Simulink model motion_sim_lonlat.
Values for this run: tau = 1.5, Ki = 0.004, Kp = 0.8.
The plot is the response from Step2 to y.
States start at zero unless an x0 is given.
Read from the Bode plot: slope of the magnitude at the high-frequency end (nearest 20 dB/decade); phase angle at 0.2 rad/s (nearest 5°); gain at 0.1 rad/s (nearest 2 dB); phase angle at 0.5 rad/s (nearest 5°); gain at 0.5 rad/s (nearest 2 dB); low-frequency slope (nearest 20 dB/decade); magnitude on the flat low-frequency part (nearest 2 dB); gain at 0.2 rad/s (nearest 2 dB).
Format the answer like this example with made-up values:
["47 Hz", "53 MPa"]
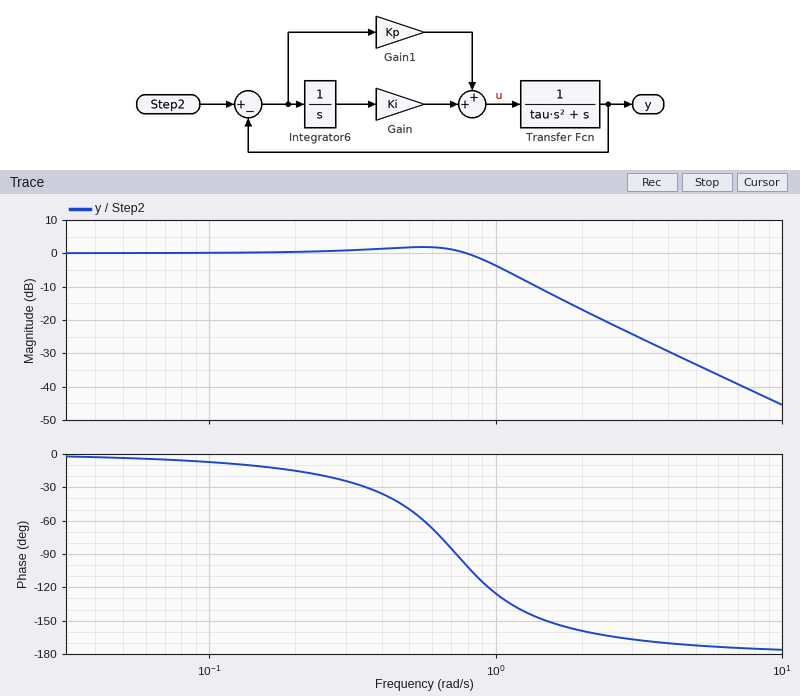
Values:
["-40 dB/decade", "-15°", "0 dB", "-50°", "2 dB", "0 dB/decade", "0 dB", "0 dB"]
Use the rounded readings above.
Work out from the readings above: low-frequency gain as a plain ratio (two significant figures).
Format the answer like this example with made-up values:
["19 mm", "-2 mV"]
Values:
["1.0"]
